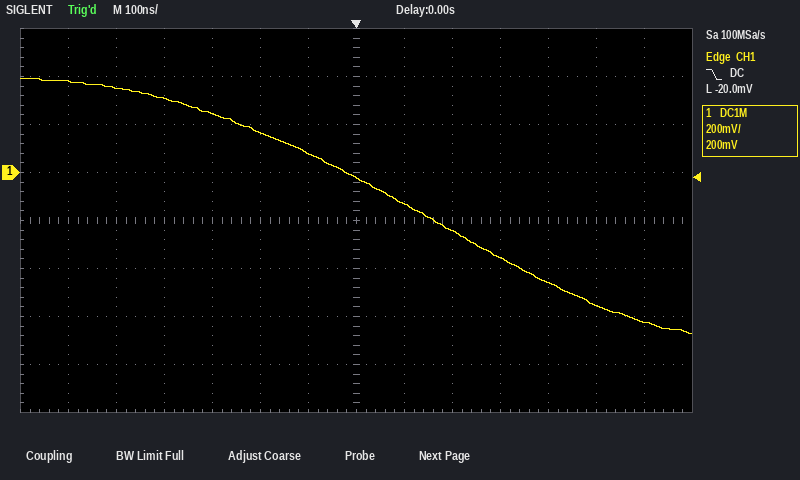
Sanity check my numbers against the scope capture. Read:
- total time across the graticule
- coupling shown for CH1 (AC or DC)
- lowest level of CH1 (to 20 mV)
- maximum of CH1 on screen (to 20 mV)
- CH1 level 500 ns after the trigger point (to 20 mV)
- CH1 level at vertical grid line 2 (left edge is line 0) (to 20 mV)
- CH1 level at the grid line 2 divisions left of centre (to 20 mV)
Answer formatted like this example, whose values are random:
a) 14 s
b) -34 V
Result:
a) 1.4 µs
b) DC
c) -680 mV
d) 400 mV
e) -560 mV
f) 360 mV
g) 160 mV
